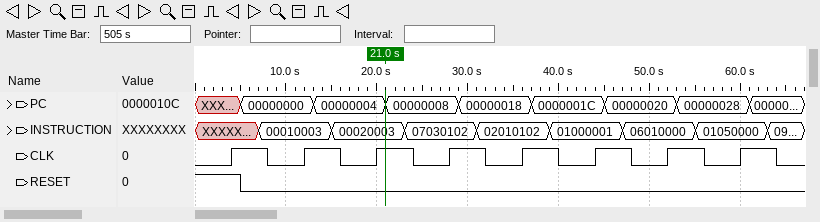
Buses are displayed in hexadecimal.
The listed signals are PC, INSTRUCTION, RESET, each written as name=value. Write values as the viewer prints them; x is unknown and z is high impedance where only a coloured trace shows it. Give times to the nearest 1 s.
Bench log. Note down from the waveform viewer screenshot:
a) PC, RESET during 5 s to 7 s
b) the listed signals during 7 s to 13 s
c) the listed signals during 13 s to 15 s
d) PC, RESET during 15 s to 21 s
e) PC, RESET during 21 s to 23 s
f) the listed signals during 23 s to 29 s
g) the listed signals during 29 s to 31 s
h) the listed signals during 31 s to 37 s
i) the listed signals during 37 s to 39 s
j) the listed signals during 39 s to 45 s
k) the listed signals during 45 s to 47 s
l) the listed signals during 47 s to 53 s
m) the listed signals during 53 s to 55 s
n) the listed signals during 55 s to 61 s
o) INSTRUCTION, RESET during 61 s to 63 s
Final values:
PC=00000000, RESET=0
PC=00000000, INSTRUCTION=00010003, RESET=0
PC=00000004, INSTRUCTION=00010003, RESET=0
PC=00000004, RESET=0
PC=00000008, RESET=0
PC=00000008, INSTRUCTION=07030102, RESET=0
PC=00000018, INSTRUCTION=07030102, RESET=0
PC=00000018, INSTRUCTION=02010102, RESET=0
PC=0000001C, INSTRUCTION=02010102, RESET=0
PC=0000001C, INSTRUCTION=01000001, RESET=0
PC=00000020, INSTRUCTION=01000001, RESET=0
PC=00000020, INSTRUCTION=06010000, RESET=0
PC=00000028, INSTRUCTION=06010000, RESET=0
PC=00000028, INSTRUCTION=01050000, RESET=0
INSTRUCTION=01050000, RESET=0
